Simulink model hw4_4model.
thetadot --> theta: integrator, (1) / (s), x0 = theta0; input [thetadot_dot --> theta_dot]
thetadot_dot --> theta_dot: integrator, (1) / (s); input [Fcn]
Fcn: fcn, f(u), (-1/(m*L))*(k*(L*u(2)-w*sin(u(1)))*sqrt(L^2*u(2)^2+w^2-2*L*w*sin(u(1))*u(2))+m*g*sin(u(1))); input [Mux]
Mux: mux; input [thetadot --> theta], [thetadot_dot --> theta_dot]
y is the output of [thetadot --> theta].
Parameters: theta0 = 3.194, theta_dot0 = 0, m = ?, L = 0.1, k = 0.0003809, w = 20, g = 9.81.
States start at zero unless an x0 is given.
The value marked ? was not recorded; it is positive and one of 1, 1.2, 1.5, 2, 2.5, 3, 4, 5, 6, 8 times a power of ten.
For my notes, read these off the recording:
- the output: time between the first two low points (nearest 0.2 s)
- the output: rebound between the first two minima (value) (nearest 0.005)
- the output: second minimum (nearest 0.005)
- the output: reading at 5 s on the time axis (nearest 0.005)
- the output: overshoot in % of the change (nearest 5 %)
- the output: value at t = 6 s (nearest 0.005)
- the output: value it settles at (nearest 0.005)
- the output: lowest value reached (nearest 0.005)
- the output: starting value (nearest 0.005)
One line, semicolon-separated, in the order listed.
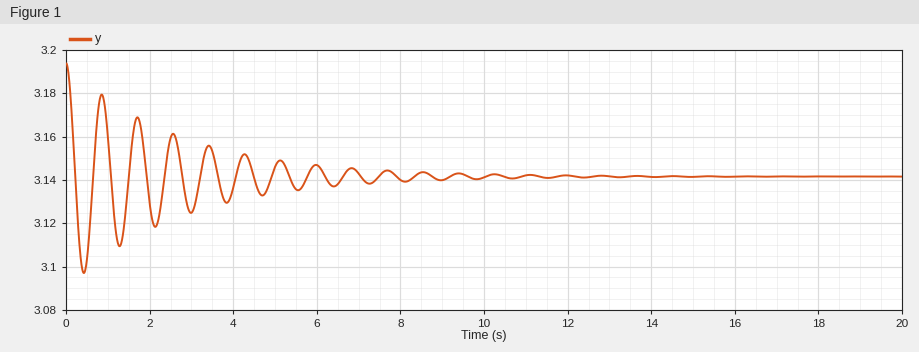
0.8 s; 3.180; 3.110; 3.145; 85 %; 3.145; 3.140; 3.095; 3.195
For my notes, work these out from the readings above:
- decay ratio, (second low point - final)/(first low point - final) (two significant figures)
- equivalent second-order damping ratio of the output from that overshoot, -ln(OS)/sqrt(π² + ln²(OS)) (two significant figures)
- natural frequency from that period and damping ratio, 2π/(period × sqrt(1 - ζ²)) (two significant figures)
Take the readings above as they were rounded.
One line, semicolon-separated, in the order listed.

0.67; 0.052; 7.9 rad/s
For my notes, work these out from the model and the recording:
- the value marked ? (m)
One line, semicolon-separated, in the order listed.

0.01
